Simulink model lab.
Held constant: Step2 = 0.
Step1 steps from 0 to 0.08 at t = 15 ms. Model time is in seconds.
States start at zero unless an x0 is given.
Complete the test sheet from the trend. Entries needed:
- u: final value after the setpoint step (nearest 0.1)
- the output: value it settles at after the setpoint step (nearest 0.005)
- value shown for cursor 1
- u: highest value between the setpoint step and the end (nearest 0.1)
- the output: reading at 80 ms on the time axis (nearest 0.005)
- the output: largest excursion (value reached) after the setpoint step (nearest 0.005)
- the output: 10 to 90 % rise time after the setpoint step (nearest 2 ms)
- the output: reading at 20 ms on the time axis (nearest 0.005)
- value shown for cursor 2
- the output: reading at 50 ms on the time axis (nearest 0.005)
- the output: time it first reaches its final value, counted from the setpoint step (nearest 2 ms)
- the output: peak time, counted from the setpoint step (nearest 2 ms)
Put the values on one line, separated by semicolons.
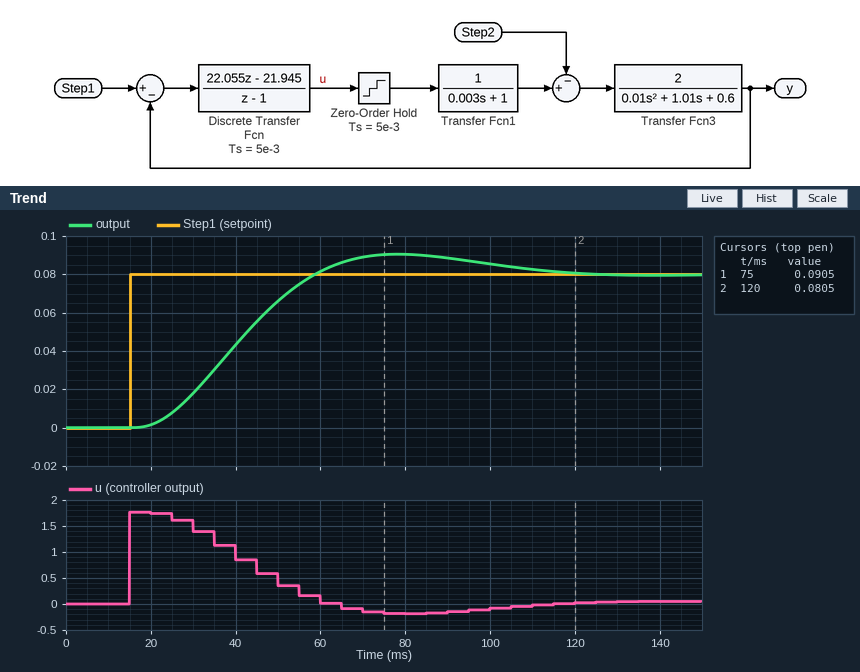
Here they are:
0.0; 0.080; 0.0905; 1.8; 0.090; 0.090; 28 ms; 0.000; 0.0805; 0.065; 44 ms; 64 ms
